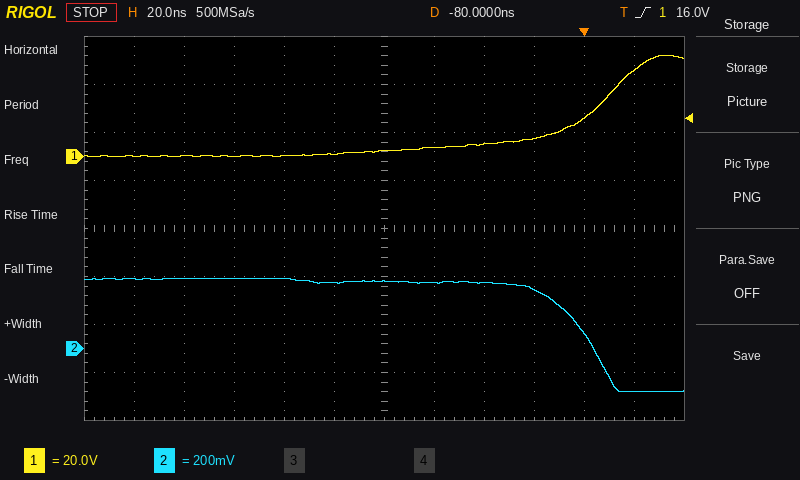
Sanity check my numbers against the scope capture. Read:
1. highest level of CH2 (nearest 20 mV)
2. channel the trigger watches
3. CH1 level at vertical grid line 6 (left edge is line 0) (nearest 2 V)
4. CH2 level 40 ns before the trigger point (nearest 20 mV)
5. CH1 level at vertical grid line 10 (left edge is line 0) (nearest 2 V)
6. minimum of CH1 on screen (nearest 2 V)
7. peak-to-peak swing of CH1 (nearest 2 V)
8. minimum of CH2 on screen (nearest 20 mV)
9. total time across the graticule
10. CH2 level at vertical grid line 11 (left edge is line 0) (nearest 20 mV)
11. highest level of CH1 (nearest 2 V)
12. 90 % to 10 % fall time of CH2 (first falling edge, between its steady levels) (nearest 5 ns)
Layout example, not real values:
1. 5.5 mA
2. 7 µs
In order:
1. 300 mV
2. CH1
3. 2 V
4. 280 mV
5. 16 V
6. 0 V
7. 42 V
8. -180 mV
9. 240 ns
10. -180 mV
11. 42 V
12. 30 ns
